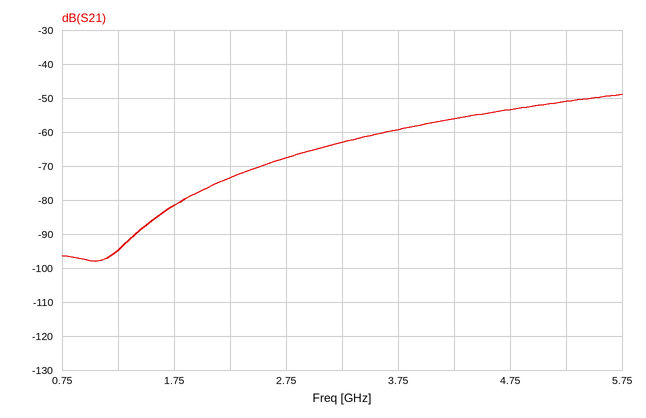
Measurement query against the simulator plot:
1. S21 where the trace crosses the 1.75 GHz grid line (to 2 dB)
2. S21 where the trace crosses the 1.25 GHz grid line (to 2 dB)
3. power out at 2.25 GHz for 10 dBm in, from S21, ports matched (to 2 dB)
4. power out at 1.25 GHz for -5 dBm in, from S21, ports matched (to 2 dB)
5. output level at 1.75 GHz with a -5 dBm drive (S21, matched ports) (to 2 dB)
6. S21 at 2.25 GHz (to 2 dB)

-82 dB
-94 dB
-64 dBm
-100 dBm
-86 dBm
-74 dB
